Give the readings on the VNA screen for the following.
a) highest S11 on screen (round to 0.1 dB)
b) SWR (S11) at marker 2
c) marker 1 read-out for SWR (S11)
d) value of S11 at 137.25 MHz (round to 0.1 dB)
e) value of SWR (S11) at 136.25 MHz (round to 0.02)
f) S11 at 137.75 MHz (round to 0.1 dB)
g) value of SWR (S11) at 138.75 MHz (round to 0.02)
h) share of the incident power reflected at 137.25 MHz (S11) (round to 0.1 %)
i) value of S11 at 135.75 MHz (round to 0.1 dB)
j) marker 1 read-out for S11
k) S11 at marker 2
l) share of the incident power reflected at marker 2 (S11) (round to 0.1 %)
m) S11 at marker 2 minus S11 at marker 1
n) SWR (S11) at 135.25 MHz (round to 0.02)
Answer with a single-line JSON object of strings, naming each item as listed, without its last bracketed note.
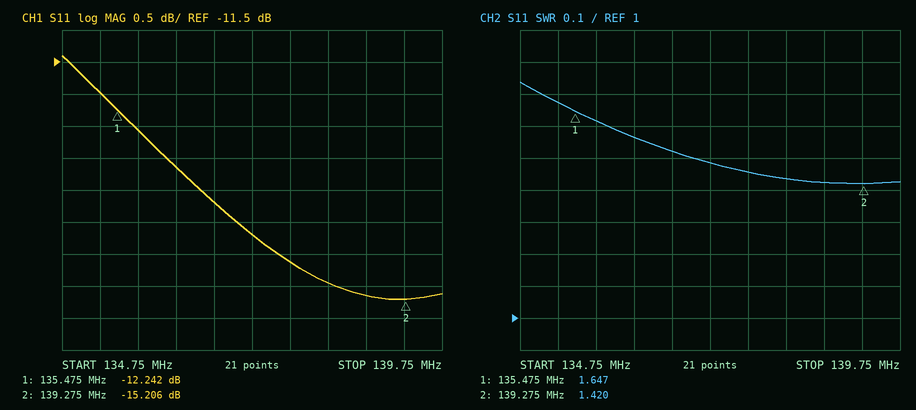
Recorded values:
{"highest S11 on screen": "-11.4 dB", "SWR (S11) at marker 2": "1.420", "marker 1 read-out for SWR": "1.647", "value of S11 at 137.25 MHz": "-14.2 dB", "value of SWR (S11) at 136.25 MHz": "1.56", "S11 at 137.75 MHz": "-14.6 dB", "value of SWR (S11) at 138.75 MHz": "1.42", "share of the incident power reflected at 137.25 MHz (S11)": "3.8 %", "value of S11 at 135.75 MHz": "-12.6 dB", "marker 1 read-out for S11": "-12.242 dB", "S11 at marker 2": "-15.206 dB", "share of the incident power reflected at marker 2 (S11)": "3.0 %", "S11 at marker 2 minus S11 at marker 1": "-2.964 dB", "SWR (S11) at 135.25 MHz": "1.68"}
